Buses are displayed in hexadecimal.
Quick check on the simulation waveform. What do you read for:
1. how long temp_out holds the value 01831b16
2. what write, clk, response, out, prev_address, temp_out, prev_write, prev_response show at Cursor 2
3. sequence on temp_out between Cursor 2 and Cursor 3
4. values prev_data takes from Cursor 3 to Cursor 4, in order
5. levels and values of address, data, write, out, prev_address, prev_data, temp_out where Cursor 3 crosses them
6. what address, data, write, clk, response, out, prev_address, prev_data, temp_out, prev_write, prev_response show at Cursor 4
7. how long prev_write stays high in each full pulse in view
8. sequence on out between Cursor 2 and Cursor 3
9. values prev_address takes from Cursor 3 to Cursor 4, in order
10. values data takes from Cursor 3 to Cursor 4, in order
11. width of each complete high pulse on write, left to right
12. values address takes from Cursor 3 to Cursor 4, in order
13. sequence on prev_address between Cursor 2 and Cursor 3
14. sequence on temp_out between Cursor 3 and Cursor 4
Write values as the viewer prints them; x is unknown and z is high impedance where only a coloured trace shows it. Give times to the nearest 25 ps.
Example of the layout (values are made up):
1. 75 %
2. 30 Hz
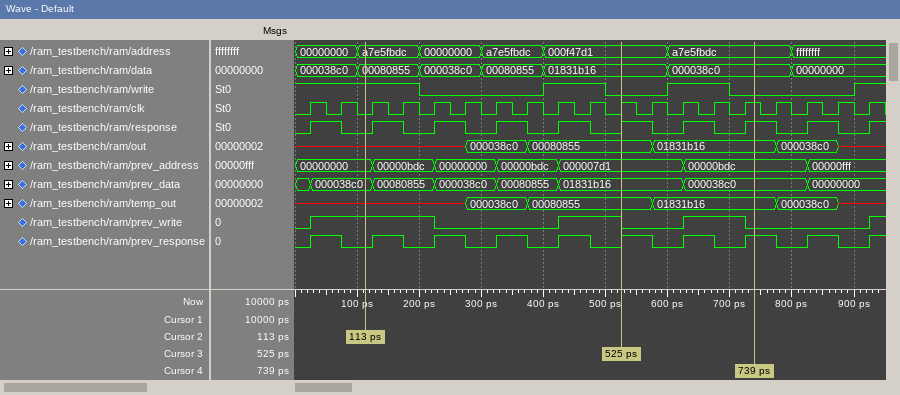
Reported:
1. 200 ps
2. write=1, clk=0, response=0, out=x, prev_address=00000000, temp_out=x, prev_write=1, prev_response=0
3. x, 000038c0, 00080855
4. 01831b16, 000038c0
5. address=000f47d1, data=01831b16, write=0, out=00080855, prev_address=000007d1, prev_data=01831b16, temp_out=00080855
6. address=a7e5fbdc, data=000038c0, write=0, clk=1, response=1, out=01831b16, prev_address=00000bdc, prev_data=000038c0, temp_out=01831b16, prev_write=0, prev_response=1
7. 200 ps, 100 ps, 100 ps
8. x, 000038c0, 00080855
9. 000007d1, 00000bdc
10. 01831b16, 000038c0
11. 100 ps, 100 ps
12. 000f47d1, a7e5fbdc
13. 00000000, 00000bdc, 00000000, 00000bdc, 000007d1
14. 00080855, 01831b16
